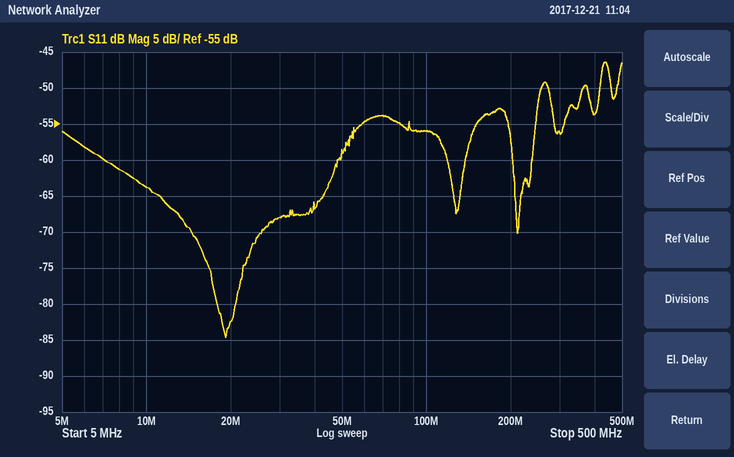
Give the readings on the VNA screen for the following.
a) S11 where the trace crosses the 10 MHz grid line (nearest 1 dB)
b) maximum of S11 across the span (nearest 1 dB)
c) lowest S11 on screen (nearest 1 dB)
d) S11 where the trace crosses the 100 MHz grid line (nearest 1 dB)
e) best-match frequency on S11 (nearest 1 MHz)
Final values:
-64 dB
-46 dB
-85 dB
-56 dB
19 MHz
